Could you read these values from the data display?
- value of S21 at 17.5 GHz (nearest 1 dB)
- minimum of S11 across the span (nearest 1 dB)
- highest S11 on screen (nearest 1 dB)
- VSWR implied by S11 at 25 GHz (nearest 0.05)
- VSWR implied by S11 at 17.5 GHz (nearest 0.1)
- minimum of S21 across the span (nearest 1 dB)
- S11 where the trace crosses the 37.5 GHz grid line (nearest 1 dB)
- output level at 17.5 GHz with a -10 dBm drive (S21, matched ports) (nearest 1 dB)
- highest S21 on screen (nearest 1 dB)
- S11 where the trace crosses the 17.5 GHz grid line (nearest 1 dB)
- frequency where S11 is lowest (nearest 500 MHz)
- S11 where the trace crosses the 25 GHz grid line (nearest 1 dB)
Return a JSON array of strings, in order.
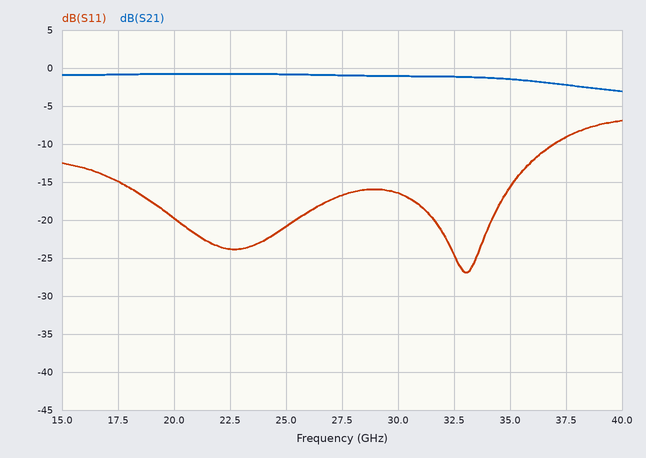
["-1 dB", "-27 dB", "-7 dB", "1.20", "1.4", "-3 dB", "-9 dB", "-11 dBm", "-1 dB", "-15 dB", "33.0 GHz", "-21 dB"]
